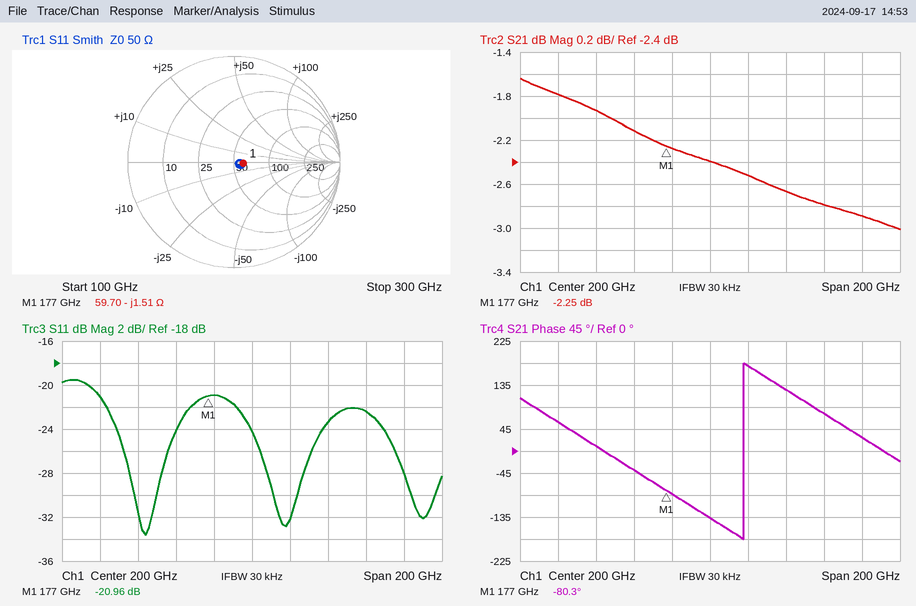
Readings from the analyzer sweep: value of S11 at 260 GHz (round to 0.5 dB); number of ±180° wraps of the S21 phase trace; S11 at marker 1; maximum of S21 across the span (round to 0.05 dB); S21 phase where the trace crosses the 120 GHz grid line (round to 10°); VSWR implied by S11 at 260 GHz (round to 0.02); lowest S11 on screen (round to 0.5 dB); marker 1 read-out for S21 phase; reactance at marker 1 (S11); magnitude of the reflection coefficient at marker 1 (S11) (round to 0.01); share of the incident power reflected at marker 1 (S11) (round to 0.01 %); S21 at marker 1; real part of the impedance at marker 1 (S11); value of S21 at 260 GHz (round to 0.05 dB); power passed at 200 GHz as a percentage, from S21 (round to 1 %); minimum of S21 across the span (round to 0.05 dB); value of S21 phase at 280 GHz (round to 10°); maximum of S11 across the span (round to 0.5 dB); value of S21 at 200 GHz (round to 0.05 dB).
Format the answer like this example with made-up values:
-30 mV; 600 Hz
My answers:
-22.5 dB; 1; -20.96 dB; -1.65 dB; 60°; 1.16; -33.5 dB; -80.3°; -1.51 Ω; 0.09; 0.80 %; -2.25 dB; 59.70 Ω; -2.80 dB; 58 %; -3.00 dB; 30°; -19.5 dB; -2.40 dB
